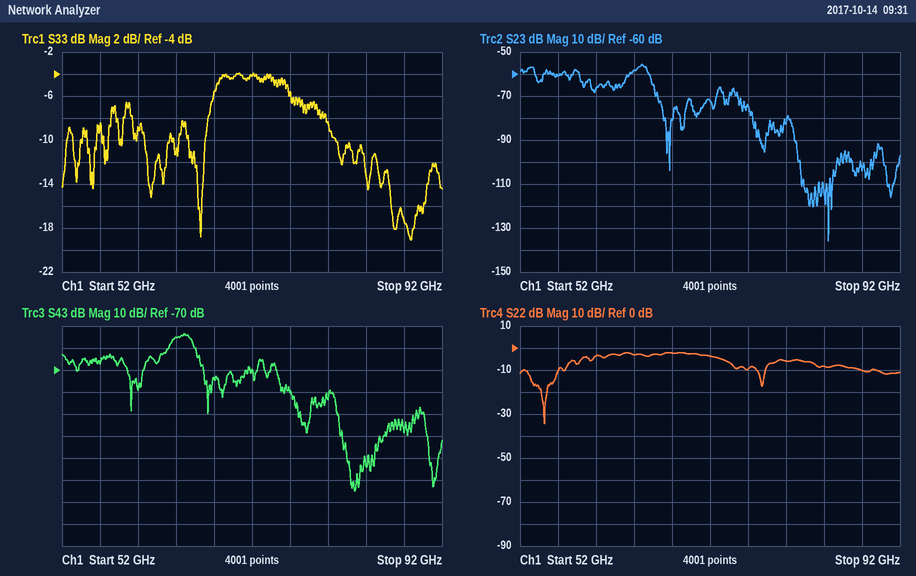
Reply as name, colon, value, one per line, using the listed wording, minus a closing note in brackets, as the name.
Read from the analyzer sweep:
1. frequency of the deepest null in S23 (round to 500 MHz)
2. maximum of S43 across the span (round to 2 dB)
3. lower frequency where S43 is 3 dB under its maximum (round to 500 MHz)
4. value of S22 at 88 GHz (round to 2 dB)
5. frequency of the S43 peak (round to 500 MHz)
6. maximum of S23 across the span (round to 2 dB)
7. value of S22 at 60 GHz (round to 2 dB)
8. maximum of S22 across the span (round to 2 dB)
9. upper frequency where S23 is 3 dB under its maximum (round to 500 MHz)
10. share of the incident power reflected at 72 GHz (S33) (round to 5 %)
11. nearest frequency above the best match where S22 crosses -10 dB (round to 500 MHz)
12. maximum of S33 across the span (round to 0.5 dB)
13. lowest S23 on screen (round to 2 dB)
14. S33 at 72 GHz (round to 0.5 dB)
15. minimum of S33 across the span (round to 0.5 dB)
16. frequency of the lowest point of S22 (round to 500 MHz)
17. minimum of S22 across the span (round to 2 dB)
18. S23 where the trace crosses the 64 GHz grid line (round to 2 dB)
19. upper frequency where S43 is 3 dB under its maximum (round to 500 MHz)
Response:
frequency of the deepest null in S23: 84.5 GHz
maximum of S43 across the span: -54 dB
lower frequency where S43 is 3 dB under its maximum: 63.5 GHz
value of S22 at 88 GHz: -10 dB
frequency of the S43 peak: 65.0 GHz
maximum of S23 across the span: -56 dB
value of S22 at 60 GHz: -4 dB
maximum of S22 across the span: -2 dB
upper frequency where S23 is 3 dB under its maximum: 65.5 GHz
share of the incident power reflected at 72 GHz (S33): 40 %
nearest frequency above the best match where S22 crosses -10 dB: 56.0 GHz
maximum of S33 across the span: -4.0 dB
lowest S23 on screen: -136 dB
S33 at 72 GHz: -4.0 dB
minimum of S33 across the span: -19.0 dB
frequency of the lowest point of S22: 54.5 GHz
minimum of S22 across the span: -34 dB
S23 where the trace crosses the 64 GHz grid line: -58 dB
upper frequency where S43 is 3 dB under its maximum: 65.5 GHz
